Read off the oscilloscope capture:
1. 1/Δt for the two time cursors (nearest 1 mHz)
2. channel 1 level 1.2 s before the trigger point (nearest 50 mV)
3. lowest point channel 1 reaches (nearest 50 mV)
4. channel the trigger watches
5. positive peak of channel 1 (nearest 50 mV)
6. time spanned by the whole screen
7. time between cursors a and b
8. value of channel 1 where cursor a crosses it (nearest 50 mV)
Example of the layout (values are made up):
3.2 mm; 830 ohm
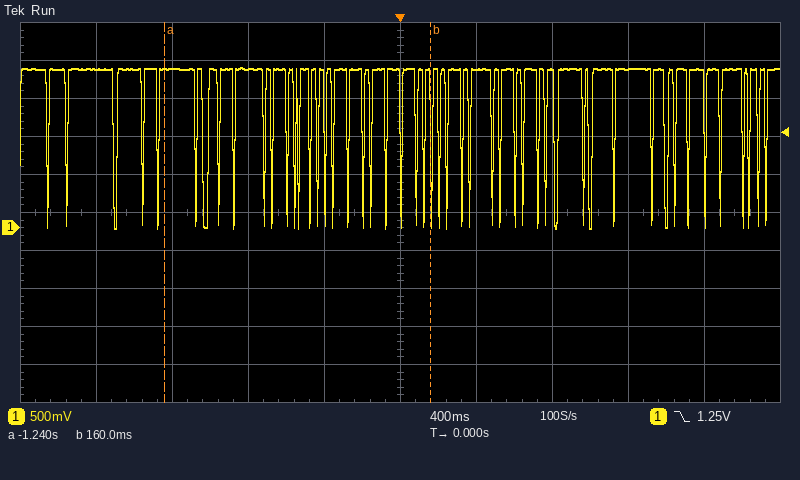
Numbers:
714 mHz; 2.10 V; 0 mV; channel 1; 2.10 V; 4 s; 1.40 s; 2.10 V
